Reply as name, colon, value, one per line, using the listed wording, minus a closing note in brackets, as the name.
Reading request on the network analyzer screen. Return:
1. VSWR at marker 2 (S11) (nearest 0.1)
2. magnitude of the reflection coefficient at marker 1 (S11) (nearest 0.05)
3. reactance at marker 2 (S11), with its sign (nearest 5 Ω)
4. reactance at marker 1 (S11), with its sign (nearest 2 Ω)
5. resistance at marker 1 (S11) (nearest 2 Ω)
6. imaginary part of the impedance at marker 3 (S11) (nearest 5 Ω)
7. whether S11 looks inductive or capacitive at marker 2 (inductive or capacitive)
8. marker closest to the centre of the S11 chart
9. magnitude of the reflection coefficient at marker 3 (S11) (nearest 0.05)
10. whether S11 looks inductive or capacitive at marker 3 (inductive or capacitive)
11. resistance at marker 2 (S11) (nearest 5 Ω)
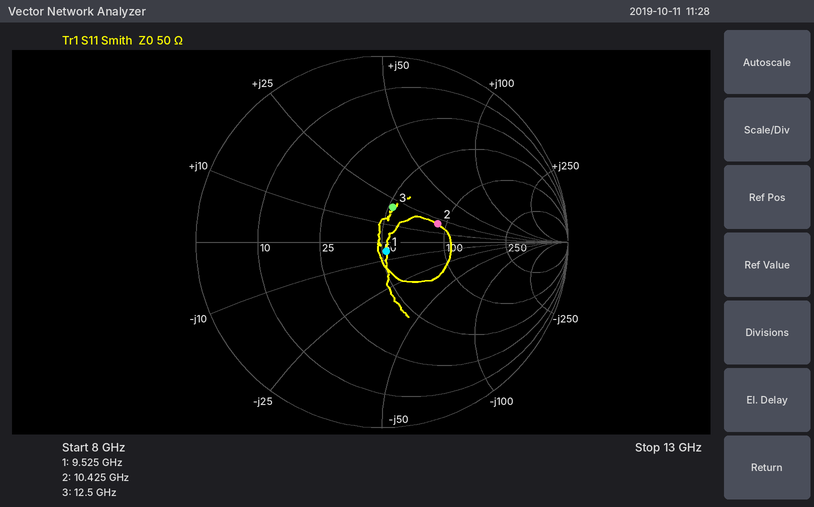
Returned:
VSWR at marker 2 (S11): 1.9
magnitude of the reflection coefficient at marker 1 (S11): 0.05
reactance at marker 2 (S11), with its sign: +20 Ω
reactance at marker 1 (S11), with its sign: -6 Ω
resistance at marker 1 (S11): 52 Ω
imaginary part of the impedance at marker 3 (S11): +20 Ω
whether S11 looks inductive or capacitive at marker 2: inductive
marker closest to the centre of the S11 chart: marker 1
magnitude of the reflection coefficient at marker 3 (S11): 0.20
whether S11 looks inductive or capacitive at marker 3: inductive
resistance at marker 2 (S11): 90 Ω
